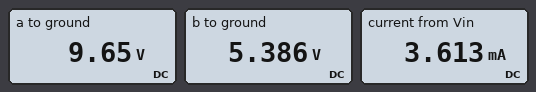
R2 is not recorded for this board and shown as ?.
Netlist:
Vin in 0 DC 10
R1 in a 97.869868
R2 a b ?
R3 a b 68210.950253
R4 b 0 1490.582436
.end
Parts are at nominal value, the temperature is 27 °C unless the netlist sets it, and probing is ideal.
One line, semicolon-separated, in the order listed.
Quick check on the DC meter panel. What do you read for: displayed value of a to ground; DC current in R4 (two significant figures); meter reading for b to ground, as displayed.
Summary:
9.65 V; 3.6 mA; 5.386 V
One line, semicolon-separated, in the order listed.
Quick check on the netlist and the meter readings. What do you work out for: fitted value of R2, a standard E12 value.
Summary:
1.2 kΩ
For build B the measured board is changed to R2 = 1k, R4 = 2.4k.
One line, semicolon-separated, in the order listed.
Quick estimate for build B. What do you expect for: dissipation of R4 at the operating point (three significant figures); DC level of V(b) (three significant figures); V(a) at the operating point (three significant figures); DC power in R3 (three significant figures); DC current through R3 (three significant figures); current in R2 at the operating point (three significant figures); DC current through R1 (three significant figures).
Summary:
19.8 mW; 6.89 V; 9.72 V; 117 µW; 41.5 µA; 2.83 mA; 2.87 mA
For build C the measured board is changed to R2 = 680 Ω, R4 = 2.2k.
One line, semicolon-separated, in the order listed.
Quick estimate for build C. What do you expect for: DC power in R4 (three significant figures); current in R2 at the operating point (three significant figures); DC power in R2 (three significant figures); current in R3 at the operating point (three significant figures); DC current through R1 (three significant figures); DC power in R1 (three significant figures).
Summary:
24.9 mW; 3.33 mA; 7.55 mW; 33.2 µA; 3.37 mA; 1.11 mW
